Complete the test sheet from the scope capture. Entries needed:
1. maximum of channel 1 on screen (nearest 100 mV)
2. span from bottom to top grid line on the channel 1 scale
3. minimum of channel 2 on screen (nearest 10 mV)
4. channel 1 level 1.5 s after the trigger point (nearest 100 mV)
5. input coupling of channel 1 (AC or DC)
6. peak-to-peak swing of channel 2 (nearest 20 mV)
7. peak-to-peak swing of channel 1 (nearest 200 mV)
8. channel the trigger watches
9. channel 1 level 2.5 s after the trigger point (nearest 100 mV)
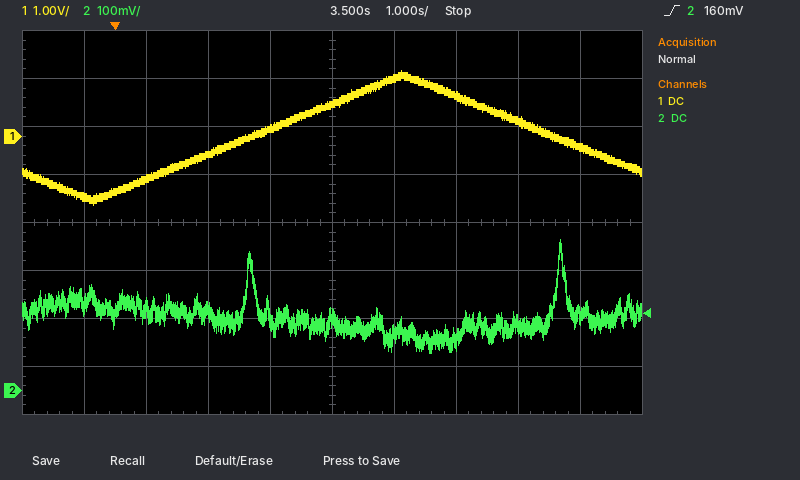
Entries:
1.4 V
8 V
80 mV
-400 mV
DC
240 mV
2.8 V
channel 2
200 mV
